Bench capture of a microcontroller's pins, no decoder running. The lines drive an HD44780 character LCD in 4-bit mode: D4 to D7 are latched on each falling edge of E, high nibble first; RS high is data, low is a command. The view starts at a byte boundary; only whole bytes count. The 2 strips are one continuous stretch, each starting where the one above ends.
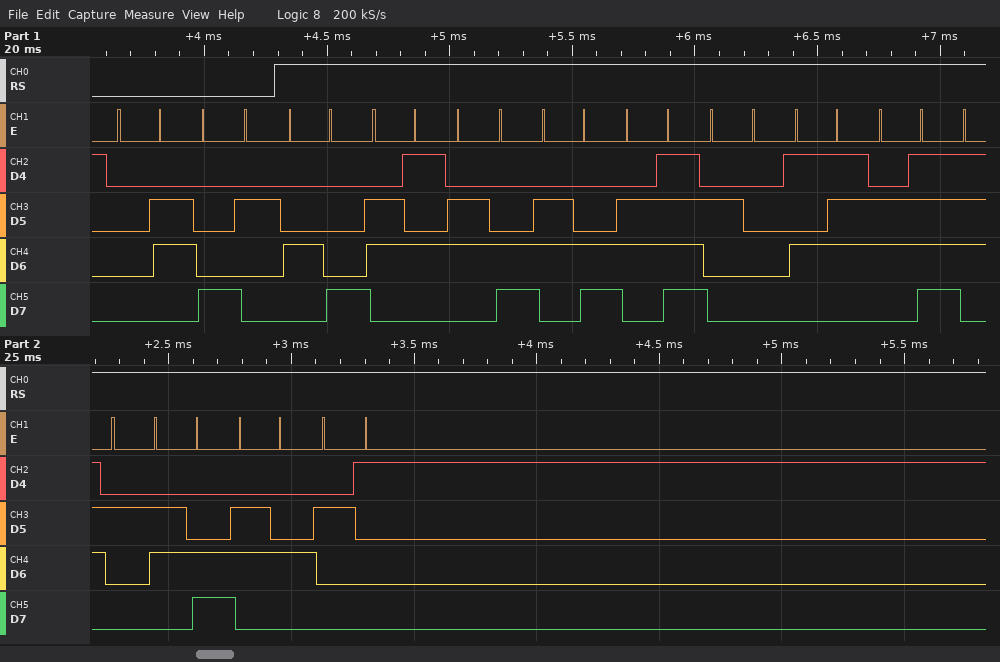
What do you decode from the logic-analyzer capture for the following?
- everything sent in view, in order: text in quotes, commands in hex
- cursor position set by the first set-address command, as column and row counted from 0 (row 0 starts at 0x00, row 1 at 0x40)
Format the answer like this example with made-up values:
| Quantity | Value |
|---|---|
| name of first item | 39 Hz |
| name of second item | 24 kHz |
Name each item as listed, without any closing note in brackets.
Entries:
| Quantity | Value |
|---|---|
| everything sent in view, in order: text in quotes, commands in hex | 0x06 0x82 "Hello World!" |
| cursor position set by the first set-address command, as column and row counted from 0 | column 2, row 0 |
